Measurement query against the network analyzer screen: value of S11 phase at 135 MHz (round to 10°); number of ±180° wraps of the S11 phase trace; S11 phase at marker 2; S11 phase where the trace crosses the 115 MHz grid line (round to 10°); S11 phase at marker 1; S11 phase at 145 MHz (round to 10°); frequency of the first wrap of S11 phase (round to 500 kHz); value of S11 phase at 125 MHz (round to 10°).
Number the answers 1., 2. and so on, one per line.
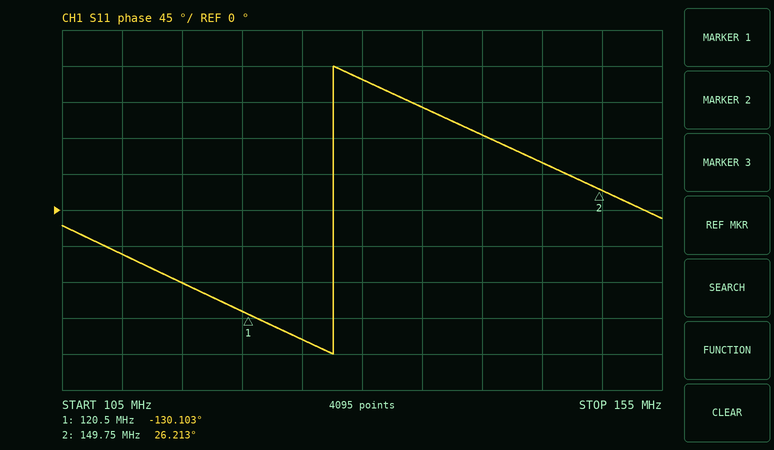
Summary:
1. 130°
2. 1
3. 26.213°
4. -90°
5. -130.103°
6. 60°
7. 127.5 MHz
8. -160°
